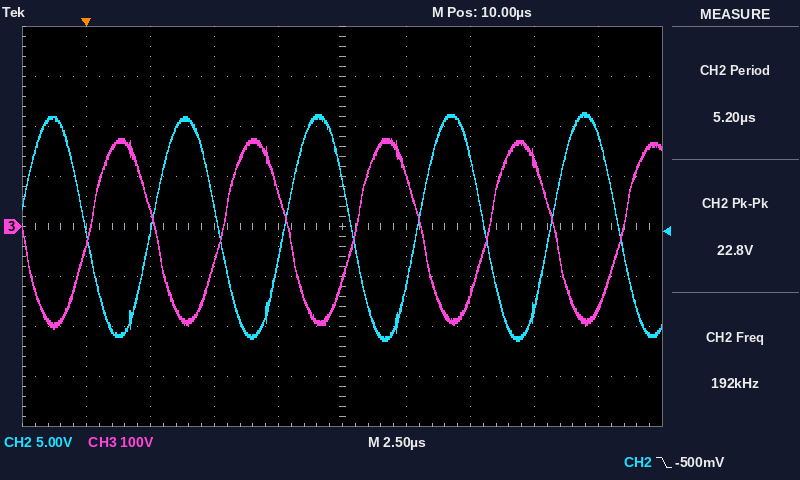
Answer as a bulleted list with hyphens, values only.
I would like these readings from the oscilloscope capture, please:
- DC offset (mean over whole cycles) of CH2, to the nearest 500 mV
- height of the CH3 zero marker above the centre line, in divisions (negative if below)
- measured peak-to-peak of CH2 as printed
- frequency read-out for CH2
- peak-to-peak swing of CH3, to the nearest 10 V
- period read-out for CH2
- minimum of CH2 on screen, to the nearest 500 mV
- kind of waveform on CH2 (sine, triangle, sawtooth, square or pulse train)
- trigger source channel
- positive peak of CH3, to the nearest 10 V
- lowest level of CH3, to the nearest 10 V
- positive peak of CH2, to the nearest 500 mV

- 0.0 V
- 0.0 div
- 22.8 V
- 192 kHz
- 380 V
- 5.20 µs
- -11.5 V
- sine
- CH2
- 180 V
- -200 V
- 11.5 V
